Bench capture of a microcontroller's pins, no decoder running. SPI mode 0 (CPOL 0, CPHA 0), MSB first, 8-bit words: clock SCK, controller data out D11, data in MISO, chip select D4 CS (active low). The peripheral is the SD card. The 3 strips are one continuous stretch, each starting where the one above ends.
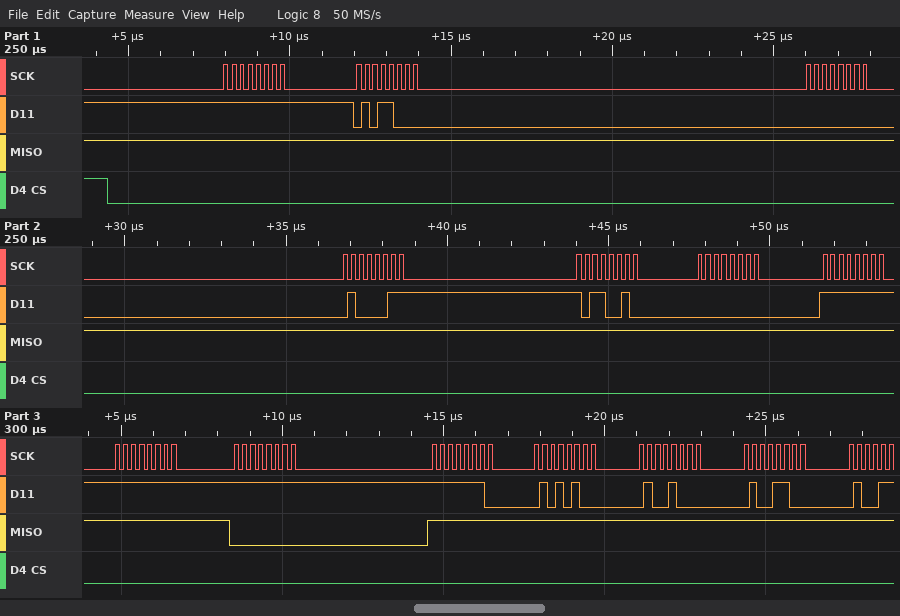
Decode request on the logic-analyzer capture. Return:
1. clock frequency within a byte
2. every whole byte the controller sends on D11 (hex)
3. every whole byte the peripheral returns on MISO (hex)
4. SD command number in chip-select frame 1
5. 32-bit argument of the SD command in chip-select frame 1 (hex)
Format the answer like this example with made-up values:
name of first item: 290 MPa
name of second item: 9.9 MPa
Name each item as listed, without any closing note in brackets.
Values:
clock frequency within a byte: 4 MHz
every whole byte the controller sends on D11: 0xFF 0x58 0x00 0x43 0xB2 0x00 0xFF 0xFF 0xFF 0xFE 0x54 0x48 0x4C
every whole byte the peripheral returns on MISO: 0xFF 0xFF 0xFF 0xFF 0xFF 0xFF 0xFF 0xFF 0x00 0xFF 0xFF 0xFF 0xFF
SD command number in chip-select frame 1: CMD24
32-bit argument of the SD command in chip-select frame 1: 0x0043B200
